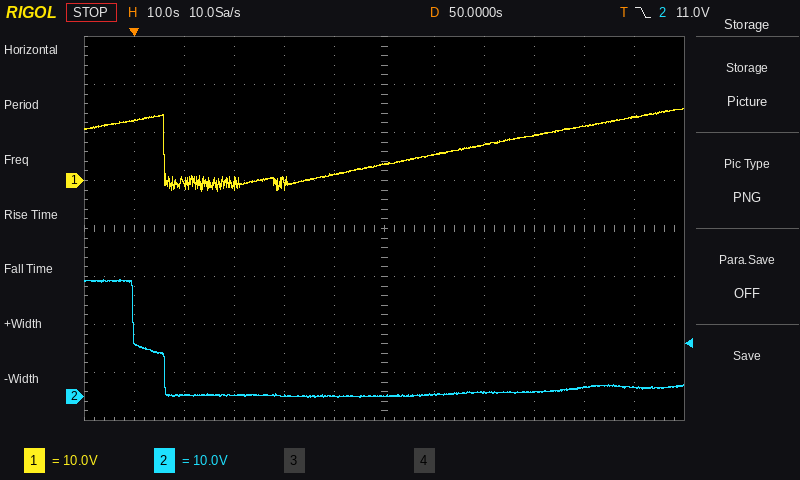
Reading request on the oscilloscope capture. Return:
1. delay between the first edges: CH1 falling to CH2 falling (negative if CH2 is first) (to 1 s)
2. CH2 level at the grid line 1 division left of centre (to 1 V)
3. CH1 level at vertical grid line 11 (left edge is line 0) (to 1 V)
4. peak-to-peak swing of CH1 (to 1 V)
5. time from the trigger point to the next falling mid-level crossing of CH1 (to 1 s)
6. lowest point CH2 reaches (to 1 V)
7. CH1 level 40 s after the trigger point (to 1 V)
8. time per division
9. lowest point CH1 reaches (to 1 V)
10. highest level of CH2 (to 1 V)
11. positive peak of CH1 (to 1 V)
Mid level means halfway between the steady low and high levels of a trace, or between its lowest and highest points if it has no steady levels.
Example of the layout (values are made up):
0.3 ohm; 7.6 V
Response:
-6 s; 0 V; 13 V; 17 V; 6 s; 0 V; 1 V; 10 s; -2 V; 24 V; 15 V
